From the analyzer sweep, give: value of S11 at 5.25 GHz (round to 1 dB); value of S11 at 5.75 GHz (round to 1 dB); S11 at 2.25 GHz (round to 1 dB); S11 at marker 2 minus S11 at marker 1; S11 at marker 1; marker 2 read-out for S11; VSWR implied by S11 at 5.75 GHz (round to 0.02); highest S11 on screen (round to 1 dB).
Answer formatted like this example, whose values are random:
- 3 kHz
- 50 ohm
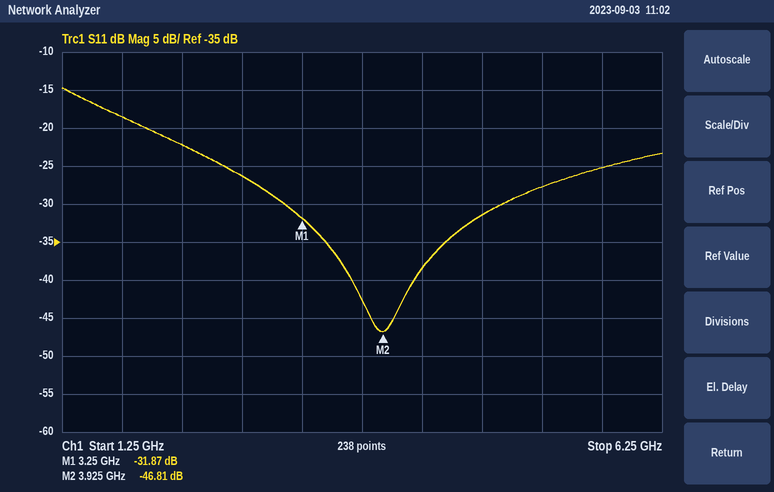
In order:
- -28 dB
- -25 dB
- -22 dB
- -14.94 dB
- -31.87 dB
- -46.81 dB
- 1.12
- -15 dB
